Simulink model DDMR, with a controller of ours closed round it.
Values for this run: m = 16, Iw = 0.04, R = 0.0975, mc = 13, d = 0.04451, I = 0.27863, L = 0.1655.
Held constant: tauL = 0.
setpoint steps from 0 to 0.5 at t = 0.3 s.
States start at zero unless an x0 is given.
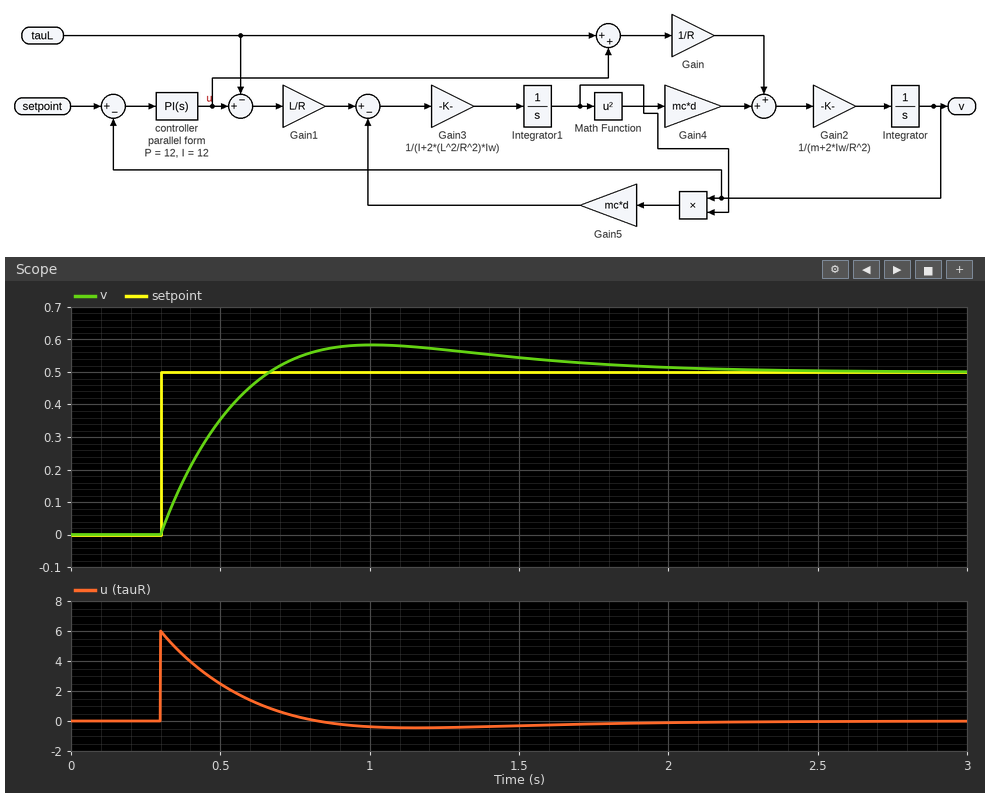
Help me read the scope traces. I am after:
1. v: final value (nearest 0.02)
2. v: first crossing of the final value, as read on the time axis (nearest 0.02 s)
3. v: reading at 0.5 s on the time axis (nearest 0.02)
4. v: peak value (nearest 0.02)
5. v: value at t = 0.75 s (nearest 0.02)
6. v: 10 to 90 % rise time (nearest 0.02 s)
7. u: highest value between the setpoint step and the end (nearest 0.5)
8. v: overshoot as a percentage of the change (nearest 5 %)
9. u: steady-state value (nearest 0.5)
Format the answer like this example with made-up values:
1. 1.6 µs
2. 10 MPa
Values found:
1. 0.50
2. 0.66 s
3. 0.36
4. 0.58
5. 0.54
6. 0.28 s
7. 6.0
8. 15 %
9. 0.0
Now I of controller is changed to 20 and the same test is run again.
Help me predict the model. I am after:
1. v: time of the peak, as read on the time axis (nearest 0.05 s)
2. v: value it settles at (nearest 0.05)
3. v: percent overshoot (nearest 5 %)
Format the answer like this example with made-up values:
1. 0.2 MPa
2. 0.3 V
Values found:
1. 0.95 s
2. 0.50
3. 20 %
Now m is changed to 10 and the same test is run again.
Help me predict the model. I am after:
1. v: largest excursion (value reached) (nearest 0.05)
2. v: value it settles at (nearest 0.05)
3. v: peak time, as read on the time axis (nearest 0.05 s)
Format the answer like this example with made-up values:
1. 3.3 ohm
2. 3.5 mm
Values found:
1. 0.55
2. 0.50
3. 0.90 s
